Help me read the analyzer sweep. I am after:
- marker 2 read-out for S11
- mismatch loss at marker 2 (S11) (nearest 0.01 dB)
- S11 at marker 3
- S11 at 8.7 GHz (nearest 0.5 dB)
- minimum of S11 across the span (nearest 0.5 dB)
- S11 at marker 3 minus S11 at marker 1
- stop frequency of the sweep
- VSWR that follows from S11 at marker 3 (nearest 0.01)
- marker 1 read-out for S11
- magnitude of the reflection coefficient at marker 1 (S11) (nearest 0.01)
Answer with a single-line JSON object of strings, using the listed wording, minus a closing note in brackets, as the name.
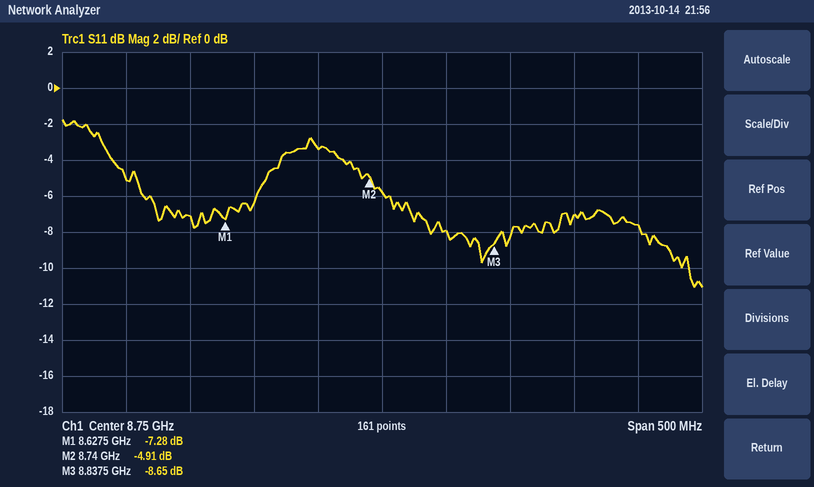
{"marker 2 read-out for S11": "-4.91 dB", "mismatch loss at marker 2 (S11)": "1.69 dB", "S11 at marker 3": "-8.65 dB", "S11 at 8.7 GHz": "-3.5 dB", "minimum of S11 across the span": "-11.0 dB", "S11 at marker 3 minus S11 at marker 1": "-1.37 dB", "stop frequency of the sweep": "9 GHz", "VSWR that follows from S11 at marker 3": "2.17", "marker 1 read-out for S11": "-7.28 dB", "magnitude of the reflection coefficient at marker 1 (S11)": "0.43"}
